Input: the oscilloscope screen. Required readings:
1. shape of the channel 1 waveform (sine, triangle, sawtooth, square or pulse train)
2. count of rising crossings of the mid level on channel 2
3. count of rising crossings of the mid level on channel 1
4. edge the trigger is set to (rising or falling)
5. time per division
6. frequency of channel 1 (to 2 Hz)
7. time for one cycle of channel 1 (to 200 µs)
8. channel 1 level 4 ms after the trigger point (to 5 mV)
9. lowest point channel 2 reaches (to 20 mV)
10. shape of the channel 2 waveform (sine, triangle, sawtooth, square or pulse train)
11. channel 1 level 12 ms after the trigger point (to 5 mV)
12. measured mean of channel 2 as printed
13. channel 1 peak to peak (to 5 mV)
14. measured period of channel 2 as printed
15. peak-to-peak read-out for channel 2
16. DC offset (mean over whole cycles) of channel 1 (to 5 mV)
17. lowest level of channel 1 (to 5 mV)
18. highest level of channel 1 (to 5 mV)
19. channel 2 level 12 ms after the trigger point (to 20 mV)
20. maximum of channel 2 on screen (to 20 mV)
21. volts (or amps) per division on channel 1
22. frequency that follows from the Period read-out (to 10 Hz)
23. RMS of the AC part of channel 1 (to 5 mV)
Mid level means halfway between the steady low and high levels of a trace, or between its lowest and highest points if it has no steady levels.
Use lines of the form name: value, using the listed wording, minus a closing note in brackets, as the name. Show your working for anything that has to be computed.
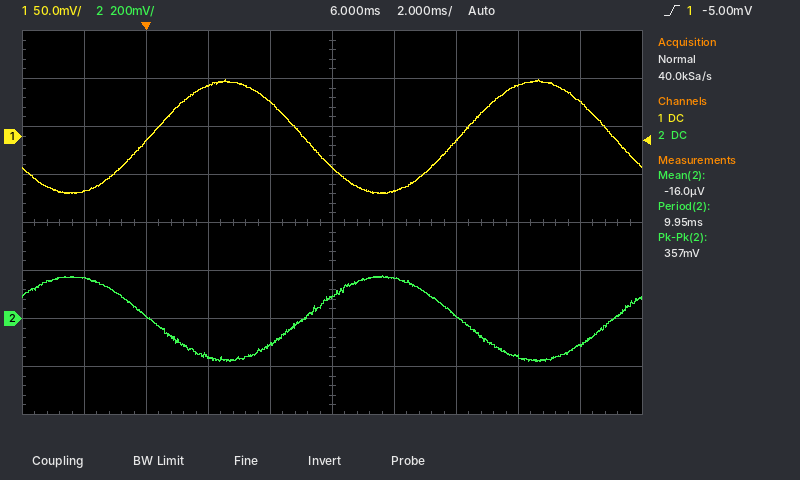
shape of the channel 1 waveform: sine
count of rising crossings of the mid level on channel 2: 2
count of rising crossings of the mid level on channel 1: 2
edge the trigger is set to: rising
time per division: 2 ms
frequency of channel 1: 1 / 10.0 ms ≈ 100 Hz
time for one cycle of channel 1: 10.0 ms
channel 1 level 4 ms after the trigger point: 35 mV
lowest point channel 2 reaches: -180 mV
shape of the channel 2 waveform: sine
channel 1 level 12 ms after the trigger point: 55 mV
measured mean of channel 2 as printed: -16.0 µV
channel 1 peak to peak: 60 mV − (-60 mV) = 120 mV
measured period of channel 2 as printed: 9.95 ms
peak-to-peak read-out for channel 2: 357 mV
DC offset (mean over whole cycles) of channel 1: (60 mV + (-60 mV)) / 2 ≈ 0 mV
lowest level of channel 1: -60 mV
highest level of channel 1: 60 mV
channel 2 level 12 ms after the trigger point: -160 mV
maximum of channel 2 on screen: 180 mV
volts (or amps) per division on channel 1: 50 mV
frequency that follows from the Period read-out: 1 / 9.95 ms ≈ 101 Hz, so 100 Hz to the nearest 10 Hz
RMS of the AC part of channel 1: 120 mV / (2√2) ≈ 42.4 mV, so 40 mV to the nearest 5 mV
